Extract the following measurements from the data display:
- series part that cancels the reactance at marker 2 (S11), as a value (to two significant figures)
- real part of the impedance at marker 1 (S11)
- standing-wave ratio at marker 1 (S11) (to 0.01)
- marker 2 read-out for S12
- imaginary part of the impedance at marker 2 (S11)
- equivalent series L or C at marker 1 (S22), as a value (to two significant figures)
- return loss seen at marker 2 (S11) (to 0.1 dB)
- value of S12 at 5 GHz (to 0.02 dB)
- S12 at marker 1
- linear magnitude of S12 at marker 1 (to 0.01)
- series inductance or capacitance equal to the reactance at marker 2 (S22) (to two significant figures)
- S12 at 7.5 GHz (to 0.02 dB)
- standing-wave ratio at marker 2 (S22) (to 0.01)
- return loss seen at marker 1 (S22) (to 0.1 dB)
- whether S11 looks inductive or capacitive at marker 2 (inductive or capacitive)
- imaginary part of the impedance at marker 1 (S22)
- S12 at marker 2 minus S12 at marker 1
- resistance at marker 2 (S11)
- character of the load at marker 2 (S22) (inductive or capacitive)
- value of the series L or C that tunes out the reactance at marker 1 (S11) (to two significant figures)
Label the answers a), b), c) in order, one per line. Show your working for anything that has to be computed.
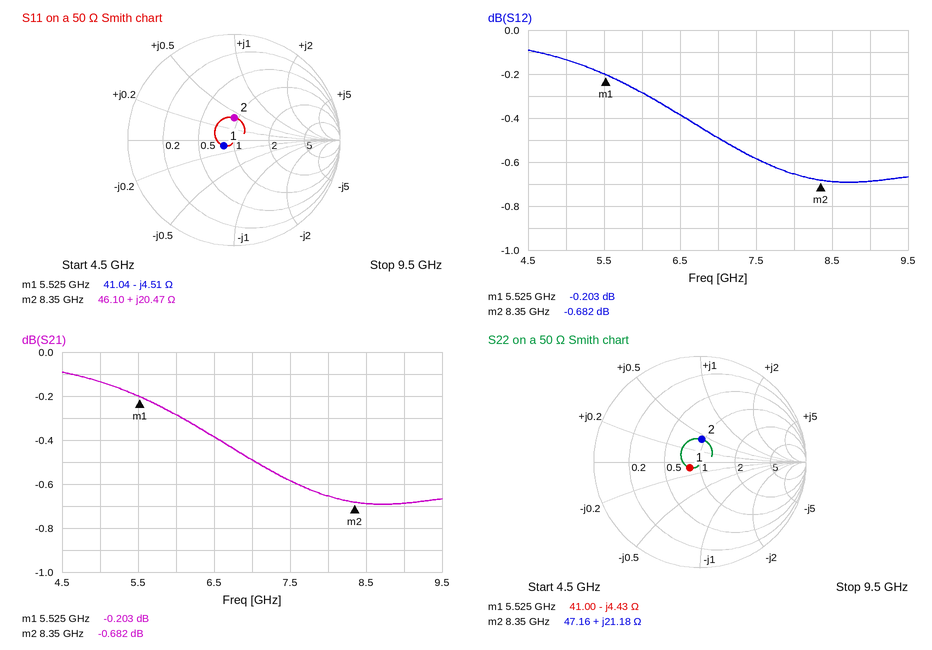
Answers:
a) C = 1/(2π × 8.35 GHz × 20.47 Ω) ≈ 931 fF, so 930 fF to two significant figures
b) 41.04 Ω
c) 1.25
d) -0.682 dB
e) +20.47 Ω
f) C = 1/(2π × 5.525 GHz × 4.43 Ω) ≈ 6.5 pF
g) 13.5 dB
h) -0.14 dB
i) -0.203 dB
j) 10^(-0.203/20) ≈ 0.98
k) L = 21.18 Ω/(2π × 8.35 GHz) ≈ 404 pH, so 400 pH to two significant figures
l) -0.58 dB
m) 1.55
n) 19.2 dB
o) inductive
p) -4.43 Ω
q) -0.682 − (-0.203) = -0.479 dB
r) 46.10 Ω
s) inductive
t) L = 4.51 Ω/(2π × 5.525 GHz) ≈ 130 pH
